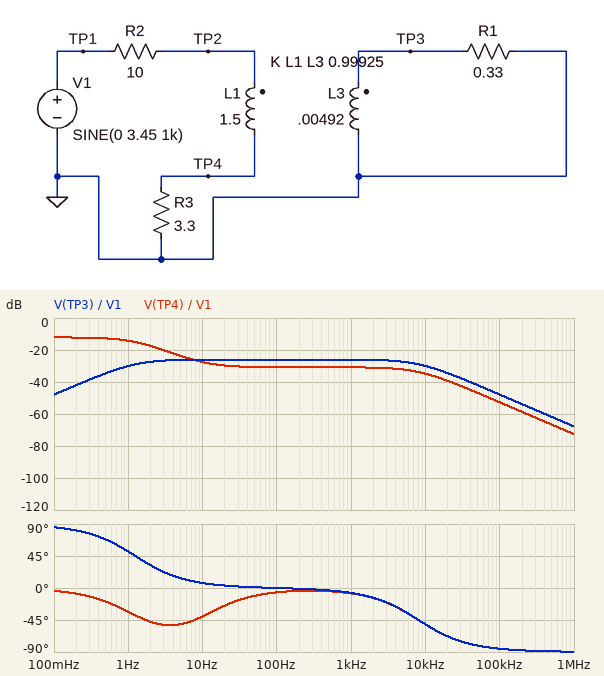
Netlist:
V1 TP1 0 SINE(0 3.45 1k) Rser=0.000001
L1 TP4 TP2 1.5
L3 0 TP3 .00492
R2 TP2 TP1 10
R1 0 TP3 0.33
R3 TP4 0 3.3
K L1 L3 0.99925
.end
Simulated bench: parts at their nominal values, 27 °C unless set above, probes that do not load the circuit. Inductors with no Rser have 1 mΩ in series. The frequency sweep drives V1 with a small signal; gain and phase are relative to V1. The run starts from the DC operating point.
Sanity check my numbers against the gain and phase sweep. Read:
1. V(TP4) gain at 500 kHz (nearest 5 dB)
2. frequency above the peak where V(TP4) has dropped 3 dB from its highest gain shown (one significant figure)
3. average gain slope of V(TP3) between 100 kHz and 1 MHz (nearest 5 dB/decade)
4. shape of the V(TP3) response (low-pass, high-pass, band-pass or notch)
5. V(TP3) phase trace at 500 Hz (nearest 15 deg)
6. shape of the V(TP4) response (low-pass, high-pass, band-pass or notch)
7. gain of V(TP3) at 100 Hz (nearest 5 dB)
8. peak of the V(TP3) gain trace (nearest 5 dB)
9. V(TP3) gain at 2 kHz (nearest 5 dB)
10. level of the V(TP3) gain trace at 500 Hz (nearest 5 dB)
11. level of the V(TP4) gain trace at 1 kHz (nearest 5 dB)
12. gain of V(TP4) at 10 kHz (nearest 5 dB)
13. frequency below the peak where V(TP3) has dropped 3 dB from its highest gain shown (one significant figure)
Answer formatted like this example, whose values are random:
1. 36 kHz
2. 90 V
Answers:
1. -65 dB
2. 1 Hz
3. -20 dB/decade
4. band-pass
5. 0 deg
6. low-pass
7. -25 dB
8. -25 dB
9. -25 dB
10. -25 dB
11. -30 dB
12. -35 dB
13. 1 Hz
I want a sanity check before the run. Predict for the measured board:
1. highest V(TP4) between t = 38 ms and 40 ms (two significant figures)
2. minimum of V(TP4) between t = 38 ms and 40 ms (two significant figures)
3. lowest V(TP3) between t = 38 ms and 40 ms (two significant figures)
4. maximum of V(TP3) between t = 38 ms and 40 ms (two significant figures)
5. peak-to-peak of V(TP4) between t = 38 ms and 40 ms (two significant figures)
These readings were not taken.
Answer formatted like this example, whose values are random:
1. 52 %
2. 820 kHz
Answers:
1. 100 mV
2. -98 mV
3. -170 mV
4. 170 mV
5. 200 mV
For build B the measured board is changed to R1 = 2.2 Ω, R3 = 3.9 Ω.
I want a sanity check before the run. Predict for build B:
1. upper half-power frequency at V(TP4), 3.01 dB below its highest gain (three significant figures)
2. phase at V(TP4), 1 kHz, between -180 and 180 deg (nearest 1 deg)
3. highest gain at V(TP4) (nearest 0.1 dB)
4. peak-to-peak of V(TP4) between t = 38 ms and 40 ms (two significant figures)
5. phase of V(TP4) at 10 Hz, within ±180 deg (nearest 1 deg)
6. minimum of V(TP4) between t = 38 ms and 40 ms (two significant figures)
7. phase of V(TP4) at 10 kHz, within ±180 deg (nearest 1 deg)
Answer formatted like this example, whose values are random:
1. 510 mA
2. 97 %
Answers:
1. 1.45 Hz
2. -5 deg
3. -11.0 dB
4. 39 mV
5. -74 deg
6. -19 mV
7. -12 deg
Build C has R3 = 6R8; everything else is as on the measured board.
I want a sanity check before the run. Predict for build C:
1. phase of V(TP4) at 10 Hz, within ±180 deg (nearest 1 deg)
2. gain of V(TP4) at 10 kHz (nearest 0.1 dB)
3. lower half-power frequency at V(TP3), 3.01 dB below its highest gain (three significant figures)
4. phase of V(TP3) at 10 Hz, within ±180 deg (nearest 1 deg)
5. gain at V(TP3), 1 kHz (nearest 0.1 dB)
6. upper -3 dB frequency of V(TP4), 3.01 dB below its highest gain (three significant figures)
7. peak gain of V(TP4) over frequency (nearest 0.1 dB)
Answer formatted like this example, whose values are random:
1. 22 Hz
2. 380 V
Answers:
1. -38 deg
2. -28.6 dB
3. 1.53 Hz
4. 9 deg
5. -26.3 dB
6. 1.56 Hz
7. -7.9 dB
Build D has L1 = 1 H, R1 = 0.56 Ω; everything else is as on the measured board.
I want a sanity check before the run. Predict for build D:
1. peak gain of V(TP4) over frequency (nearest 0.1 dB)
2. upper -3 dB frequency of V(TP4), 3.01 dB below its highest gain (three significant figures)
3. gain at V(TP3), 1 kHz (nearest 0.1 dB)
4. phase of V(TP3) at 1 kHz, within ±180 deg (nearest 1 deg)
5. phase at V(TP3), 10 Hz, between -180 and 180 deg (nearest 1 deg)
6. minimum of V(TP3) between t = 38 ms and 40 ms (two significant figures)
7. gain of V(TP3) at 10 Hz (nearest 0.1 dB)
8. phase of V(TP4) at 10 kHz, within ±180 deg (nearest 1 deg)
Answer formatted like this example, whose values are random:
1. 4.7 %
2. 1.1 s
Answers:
1. -12.1 dB
2. 1.92 Hz
3. -24.1 dB
4. -4 deg
5. 11 deg
6. -220 mV
7. -24.2 dB
8. -37 deg
